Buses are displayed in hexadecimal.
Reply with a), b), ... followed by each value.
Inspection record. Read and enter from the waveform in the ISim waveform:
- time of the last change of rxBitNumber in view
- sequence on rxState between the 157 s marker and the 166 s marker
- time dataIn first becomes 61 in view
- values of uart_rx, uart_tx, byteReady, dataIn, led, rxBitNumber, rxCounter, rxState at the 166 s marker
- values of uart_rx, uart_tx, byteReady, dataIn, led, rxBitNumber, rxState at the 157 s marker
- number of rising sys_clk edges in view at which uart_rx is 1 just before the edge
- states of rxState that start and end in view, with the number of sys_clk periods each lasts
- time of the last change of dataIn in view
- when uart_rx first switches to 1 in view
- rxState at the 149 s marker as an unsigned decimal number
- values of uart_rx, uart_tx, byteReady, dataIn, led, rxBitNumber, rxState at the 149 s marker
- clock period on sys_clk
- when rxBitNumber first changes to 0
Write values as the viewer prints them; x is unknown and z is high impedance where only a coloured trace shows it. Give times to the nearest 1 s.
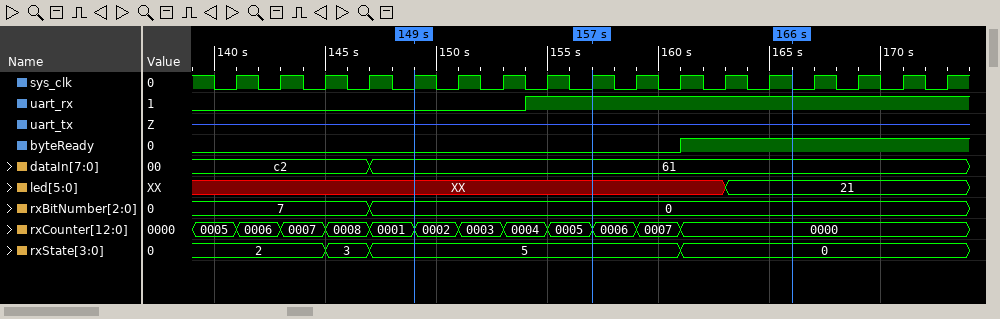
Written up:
a) 147 s
b) 5, 0
c) 147 s
d) uart_rx=1, uart_tx=z, byteReady=1, dataIn=61, led=21, rxBitNumber=0, rxCounter=0000, rxState=0
e) uart_rx=1, uart_tx=z, byteReady=0, dataIn=61, led=XX, rxBitNumber=0, rxState=5
f) 10
g) 3: 1, 5: 7
h) 147 s
i) 154 s
j) 5
k) uart_rx=0, uart_tx=z, byteReady=0, dataIn=61, led=XX, rxBitNumber=0, rxState=5
l) 2 s
m) 147 s
